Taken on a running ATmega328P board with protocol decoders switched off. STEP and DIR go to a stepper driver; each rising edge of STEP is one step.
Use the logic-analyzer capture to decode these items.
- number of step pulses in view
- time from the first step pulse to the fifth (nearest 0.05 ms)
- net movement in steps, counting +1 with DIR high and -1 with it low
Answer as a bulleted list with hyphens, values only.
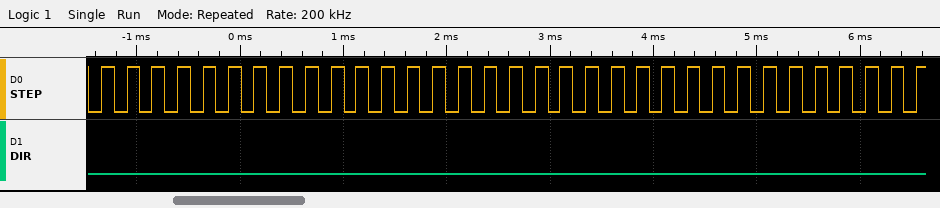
- 33
- 1.00 ms
- -33
